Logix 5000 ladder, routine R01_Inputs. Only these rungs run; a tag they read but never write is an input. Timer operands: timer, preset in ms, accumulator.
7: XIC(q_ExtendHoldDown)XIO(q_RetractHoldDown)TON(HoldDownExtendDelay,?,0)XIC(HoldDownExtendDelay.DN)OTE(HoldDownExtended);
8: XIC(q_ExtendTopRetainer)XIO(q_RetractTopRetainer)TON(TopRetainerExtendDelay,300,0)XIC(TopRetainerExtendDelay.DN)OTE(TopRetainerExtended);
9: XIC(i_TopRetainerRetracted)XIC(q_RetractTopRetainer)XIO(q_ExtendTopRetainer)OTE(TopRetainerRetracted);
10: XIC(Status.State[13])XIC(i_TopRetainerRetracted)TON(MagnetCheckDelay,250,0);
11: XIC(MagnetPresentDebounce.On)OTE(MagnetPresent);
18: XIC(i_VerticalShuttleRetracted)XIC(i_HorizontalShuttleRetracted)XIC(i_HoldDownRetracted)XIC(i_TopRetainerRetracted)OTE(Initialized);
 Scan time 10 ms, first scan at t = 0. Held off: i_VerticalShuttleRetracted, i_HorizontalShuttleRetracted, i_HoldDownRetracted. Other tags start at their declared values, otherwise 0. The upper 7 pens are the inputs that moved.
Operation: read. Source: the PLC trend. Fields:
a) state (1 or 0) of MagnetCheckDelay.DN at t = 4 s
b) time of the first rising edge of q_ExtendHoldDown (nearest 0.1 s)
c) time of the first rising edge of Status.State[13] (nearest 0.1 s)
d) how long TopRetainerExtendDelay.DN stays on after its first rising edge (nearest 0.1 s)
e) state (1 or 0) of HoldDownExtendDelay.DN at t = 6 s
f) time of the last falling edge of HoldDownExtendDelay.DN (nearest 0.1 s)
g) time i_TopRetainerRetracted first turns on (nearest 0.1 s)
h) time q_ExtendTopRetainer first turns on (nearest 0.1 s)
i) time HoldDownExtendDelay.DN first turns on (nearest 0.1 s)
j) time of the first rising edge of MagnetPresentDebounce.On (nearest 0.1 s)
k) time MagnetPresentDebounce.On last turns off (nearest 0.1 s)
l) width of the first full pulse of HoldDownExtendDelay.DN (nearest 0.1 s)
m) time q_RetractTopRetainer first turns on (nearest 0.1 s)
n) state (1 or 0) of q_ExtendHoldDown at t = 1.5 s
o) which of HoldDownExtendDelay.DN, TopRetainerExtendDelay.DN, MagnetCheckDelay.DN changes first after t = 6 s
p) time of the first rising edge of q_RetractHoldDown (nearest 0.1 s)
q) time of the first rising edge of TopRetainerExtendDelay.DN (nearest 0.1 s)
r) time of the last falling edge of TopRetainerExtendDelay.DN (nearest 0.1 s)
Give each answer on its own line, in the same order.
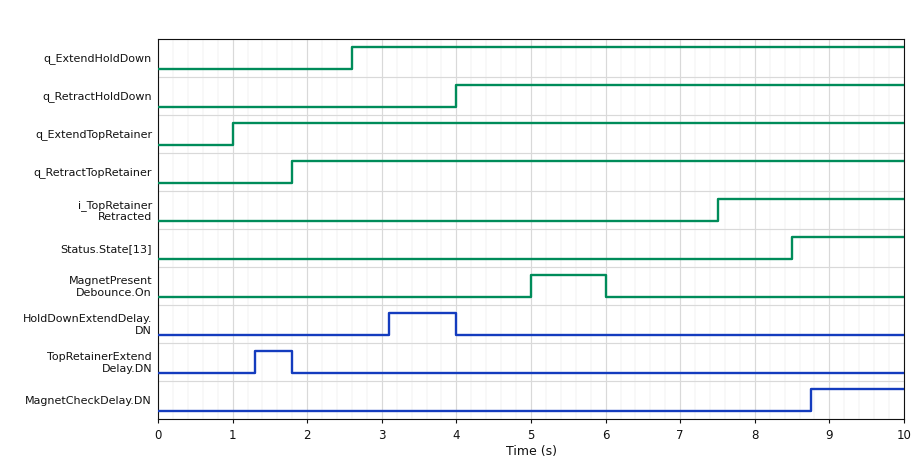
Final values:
0
2.6 s
8.5 s
0.5 s
0
4.0 s
7.5 s
1.0 s
3.1 s
5.0 s
6.0 s
0.9 s
1.8 s
0
MagnetCheckDelay.DN
4.0 s
1.3 s
1.8 s
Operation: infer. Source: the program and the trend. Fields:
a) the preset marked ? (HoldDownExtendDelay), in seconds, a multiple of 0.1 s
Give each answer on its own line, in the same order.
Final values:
0.5 s
